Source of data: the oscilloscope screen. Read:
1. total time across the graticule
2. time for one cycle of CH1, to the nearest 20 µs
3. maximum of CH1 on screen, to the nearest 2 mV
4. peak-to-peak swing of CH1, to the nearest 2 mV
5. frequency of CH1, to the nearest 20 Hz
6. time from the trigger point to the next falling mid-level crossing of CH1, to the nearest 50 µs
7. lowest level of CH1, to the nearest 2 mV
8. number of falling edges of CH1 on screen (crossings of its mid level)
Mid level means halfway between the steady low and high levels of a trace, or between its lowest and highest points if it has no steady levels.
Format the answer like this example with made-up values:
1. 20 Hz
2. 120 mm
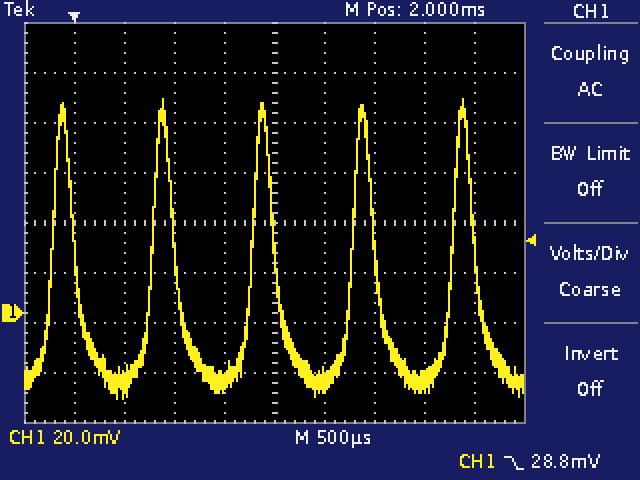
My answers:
1. 5 ms
2. 1.00 ms
3. 86 mV
4. 120 mV
5. 1.00 kHz
6. 1.00 ms
7. -34 mV
8. 5
